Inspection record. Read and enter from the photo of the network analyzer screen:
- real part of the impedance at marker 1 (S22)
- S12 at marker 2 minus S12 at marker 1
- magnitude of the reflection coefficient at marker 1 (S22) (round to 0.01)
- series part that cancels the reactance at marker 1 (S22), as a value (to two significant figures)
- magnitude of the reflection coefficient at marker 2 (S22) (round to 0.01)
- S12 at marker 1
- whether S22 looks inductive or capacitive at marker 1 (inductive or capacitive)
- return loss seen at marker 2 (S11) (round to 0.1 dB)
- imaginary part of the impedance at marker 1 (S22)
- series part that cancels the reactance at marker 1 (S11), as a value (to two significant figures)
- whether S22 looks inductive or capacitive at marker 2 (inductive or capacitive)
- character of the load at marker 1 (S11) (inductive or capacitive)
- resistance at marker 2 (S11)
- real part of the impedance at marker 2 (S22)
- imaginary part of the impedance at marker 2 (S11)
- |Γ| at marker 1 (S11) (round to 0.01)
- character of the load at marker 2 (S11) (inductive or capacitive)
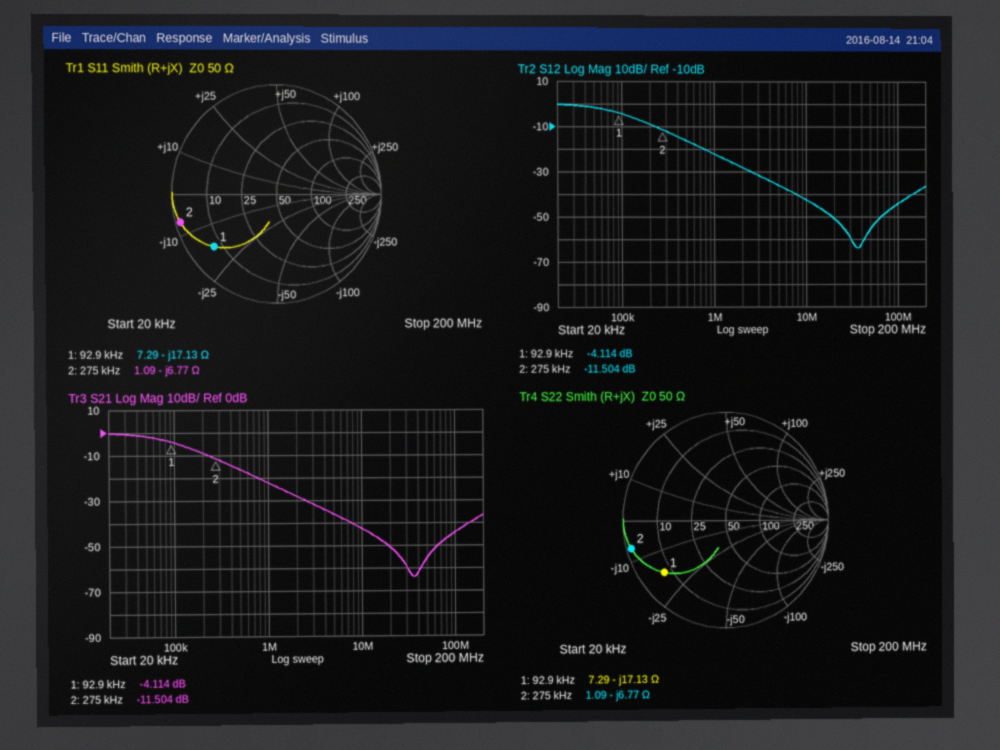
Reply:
7.29 Ω
-7.390 dB
0.77
29 µH
0.96
-4.114 dB
capacitive
0.4 dB
-17.13 Ω
29 µH
capacitive
capacitive
1.09 Ω
1.09 Ω
-6.77 Ω
0.77
capacitive
